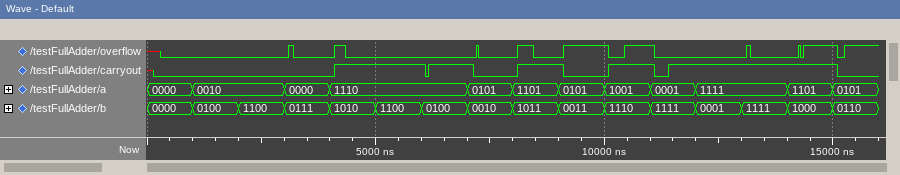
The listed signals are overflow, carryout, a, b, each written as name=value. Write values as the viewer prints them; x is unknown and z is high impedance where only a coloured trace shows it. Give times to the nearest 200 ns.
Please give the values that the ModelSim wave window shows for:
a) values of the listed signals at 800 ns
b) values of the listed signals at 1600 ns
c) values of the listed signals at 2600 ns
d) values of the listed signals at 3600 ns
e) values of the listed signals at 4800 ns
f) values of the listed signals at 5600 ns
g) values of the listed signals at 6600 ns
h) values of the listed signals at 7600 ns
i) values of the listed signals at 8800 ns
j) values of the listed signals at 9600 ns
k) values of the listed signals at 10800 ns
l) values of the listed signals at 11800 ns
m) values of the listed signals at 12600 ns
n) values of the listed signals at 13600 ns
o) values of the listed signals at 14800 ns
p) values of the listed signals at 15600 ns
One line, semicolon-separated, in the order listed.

overflow=0, carryout=0, a=0000, b=0000; overflow=0, carryout=0, a=0010, b=0100; overflow=0, carryout=0, a=0010, b=1100; overflow=0, carryout=0, a=0000, b=0111; overflow=0, carryout=1, a=1110, b=1010; overflow=0, carryout=1, a=1110, b=1100; overflow=0, carryout=1, a=1110, b=0100; overflow=0, carryout=0, a=0101, b=0010; overflow=0, carryout=1, a=1101, b=1011; overflow=1, carryout=0, a=0101, b=0011; overflow=1, carryout=1, a=1001, b=1110; overflow=0, carryout=1, a=0001, b=1111; overflow=0, carryout=1, a=1111, b=0001; overflow=0, carryout=1, a=1111, b=1111; overflow=1, carryout=1, a=1101, b=1000; overflow=1, carryout=0, a=0101, b=0110
